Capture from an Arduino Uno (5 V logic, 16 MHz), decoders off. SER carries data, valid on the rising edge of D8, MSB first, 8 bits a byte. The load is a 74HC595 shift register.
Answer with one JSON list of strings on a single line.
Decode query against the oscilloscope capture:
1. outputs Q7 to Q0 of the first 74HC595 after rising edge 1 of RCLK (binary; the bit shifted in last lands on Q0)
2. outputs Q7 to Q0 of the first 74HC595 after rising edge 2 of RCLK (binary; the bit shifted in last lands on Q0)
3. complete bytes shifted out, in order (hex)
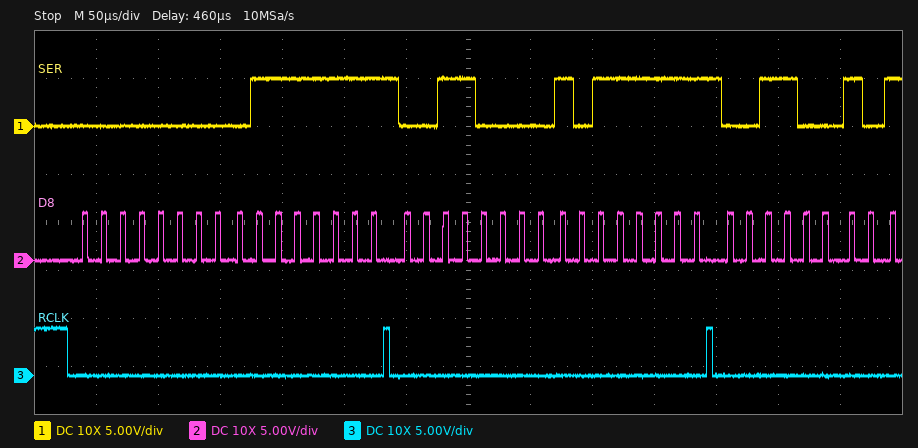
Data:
["01111111", "10111111", "00 7F 30 BF 32"]
